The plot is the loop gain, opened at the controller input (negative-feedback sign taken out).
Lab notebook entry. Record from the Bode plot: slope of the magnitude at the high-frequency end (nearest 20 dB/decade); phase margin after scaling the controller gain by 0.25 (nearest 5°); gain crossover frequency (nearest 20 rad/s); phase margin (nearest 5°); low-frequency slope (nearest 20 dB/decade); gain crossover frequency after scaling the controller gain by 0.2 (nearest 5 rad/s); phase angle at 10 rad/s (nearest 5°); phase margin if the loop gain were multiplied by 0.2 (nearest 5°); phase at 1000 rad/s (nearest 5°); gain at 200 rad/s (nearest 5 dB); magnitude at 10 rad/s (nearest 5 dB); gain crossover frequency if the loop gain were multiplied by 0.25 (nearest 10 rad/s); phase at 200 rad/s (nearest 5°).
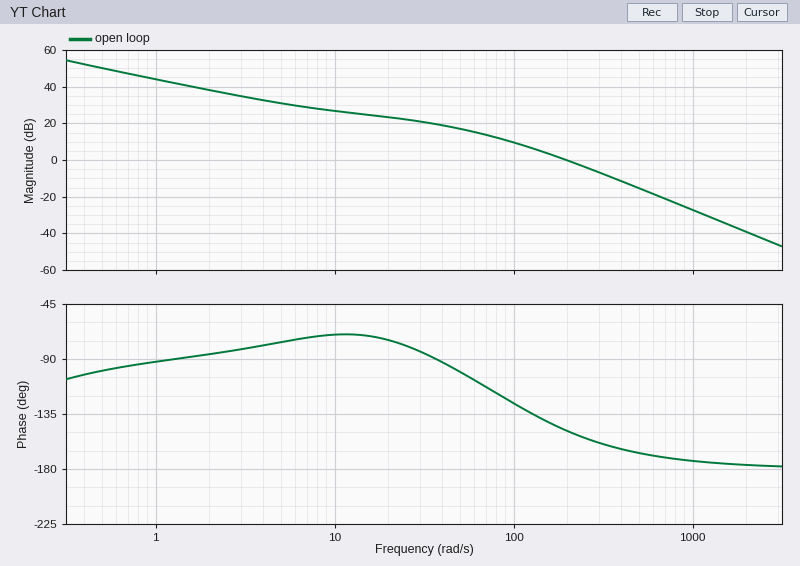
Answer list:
-40 dB/decade
60°
200 rad/s
30°
-20 dB/decade
70 rad/s
-70°
70°
-175°
0 dB
25 dB
80 rad/s
-150°
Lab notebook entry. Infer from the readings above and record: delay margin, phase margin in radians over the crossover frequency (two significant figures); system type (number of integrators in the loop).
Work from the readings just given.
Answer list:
0.0026 s
1
